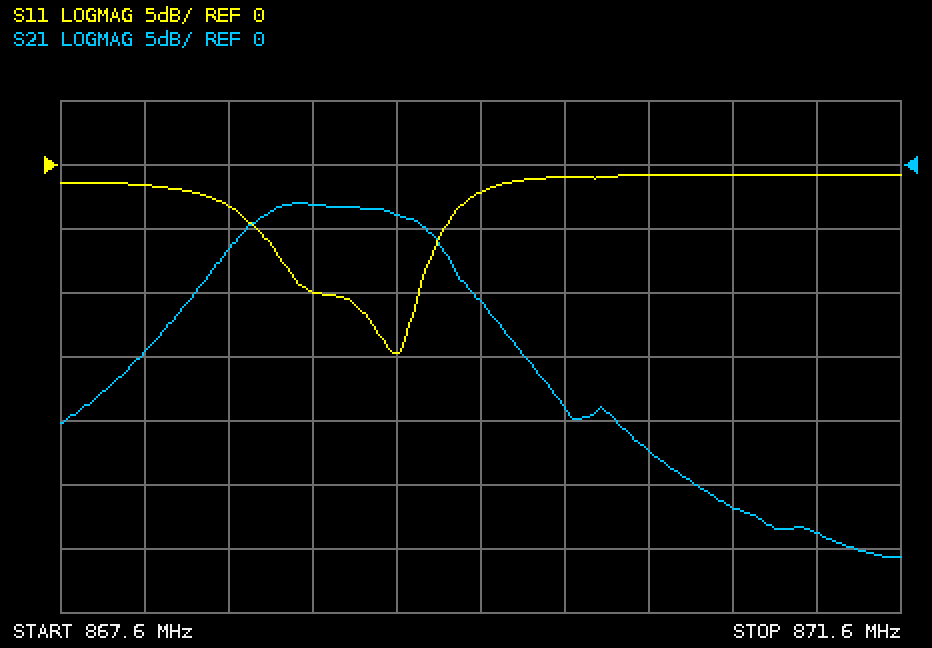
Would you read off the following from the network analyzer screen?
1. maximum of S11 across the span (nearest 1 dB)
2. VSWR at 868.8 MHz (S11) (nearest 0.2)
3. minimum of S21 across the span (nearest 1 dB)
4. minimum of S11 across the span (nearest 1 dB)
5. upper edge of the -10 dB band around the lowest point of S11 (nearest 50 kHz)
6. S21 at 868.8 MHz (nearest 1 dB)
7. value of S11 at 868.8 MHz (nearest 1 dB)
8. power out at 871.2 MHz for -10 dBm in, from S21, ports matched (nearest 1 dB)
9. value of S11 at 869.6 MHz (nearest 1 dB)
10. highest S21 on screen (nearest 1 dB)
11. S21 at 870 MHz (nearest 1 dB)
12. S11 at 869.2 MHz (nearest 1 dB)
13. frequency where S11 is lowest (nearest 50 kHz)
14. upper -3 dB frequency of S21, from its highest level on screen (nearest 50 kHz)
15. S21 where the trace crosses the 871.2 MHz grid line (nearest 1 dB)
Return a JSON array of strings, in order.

["-1 dB", "2.0", "-31 dB", "-15 dB", "869.30 MHz", "-3 dB", "-10 dB", "-39 dBm", "-2 dB", "-3 dB", "-19 dB", "-15 dB", "869.20 MHz", "869.40 MHz", "-29 dB"]
